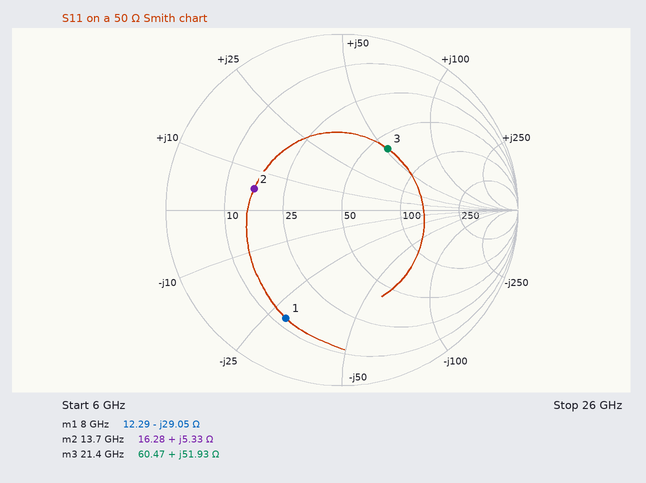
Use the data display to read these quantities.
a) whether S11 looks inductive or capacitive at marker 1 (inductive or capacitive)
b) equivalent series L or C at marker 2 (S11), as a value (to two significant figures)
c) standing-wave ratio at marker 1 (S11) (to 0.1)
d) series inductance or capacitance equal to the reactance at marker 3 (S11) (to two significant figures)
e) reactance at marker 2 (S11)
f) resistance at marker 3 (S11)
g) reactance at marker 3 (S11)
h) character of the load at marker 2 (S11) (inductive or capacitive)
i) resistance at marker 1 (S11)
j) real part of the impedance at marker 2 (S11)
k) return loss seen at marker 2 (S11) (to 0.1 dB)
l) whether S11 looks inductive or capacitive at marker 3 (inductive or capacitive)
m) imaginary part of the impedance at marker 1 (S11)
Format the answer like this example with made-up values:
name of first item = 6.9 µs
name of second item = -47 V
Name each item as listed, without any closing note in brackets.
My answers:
whether S11 looks inductive or capacitive at marker 1 = capacitive
equivalent series L or C at marker 2 (S11), as a value = 62 pH
standing-wave ratio at marker 1 (S11) = 5.5
series inductance or capacitance equal to the reactance at marker 3 (S11) = 390 pH
reactance at marker 2 = +5.33 Ω
resistance at marker 3 = 60.47 Ω
reactance at marker 3 = +51.93 Ω
character of the load at marker 2 (S11) = inductive
resistance at marker 1 = 12.29 Ω
real part of the impedance at marker 2 = 16.28 Ω
return loss seen at marker 2 (S11) = 5.8 dB
whether S11 looks inductive or capacitive at marker 3 = inductive
imaginary part of the impedance at marker 1 = -29.05 Ω
